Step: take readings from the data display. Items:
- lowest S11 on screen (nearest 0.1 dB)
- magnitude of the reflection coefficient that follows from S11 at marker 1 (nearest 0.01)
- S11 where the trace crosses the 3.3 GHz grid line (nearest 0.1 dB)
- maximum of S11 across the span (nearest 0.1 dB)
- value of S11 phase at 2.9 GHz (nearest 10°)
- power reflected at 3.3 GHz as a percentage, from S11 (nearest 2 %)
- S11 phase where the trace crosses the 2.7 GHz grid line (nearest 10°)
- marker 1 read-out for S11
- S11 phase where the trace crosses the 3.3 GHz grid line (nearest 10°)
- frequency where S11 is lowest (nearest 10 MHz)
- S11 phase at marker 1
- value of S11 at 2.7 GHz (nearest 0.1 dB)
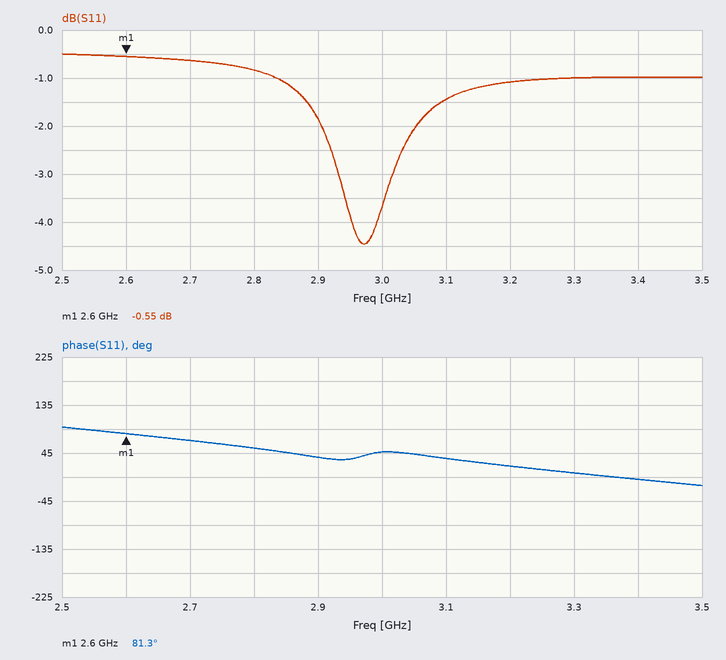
-4.5 dB
0.94
-1.0 dB
-0.5 dB
40°
80 %
70°
-0.55 dB
10°
2.97 GHz
81.3°
-0.6 dB
